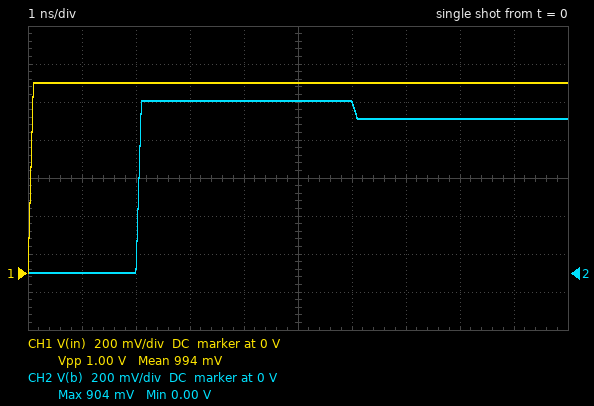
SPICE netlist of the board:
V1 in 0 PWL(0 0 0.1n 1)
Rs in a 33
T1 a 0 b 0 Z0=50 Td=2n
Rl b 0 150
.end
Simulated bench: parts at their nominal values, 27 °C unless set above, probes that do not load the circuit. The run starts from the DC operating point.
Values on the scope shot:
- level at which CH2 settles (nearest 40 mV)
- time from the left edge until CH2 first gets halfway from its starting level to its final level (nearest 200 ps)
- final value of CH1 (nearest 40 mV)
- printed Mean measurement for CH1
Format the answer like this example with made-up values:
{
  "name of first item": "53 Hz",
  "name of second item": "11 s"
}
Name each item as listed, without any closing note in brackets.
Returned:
{
  "level at which CH2 settles": "800 mV",
  "time from the left edge until CH2 first gets halfway from its starting level to its final level": "2.0 ns",
  "final value of CH1": "1.00 V",
  "printed Mean measurement for CH1": "994 mV"
}
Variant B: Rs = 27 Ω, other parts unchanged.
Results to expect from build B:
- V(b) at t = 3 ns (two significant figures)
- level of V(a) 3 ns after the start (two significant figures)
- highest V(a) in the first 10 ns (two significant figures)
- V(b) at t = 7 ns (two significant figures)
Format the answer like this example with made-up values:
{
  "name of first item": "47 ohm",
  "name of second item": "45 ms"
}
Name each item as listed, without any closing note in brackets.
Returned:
{
  "V(b) at t = 3 ns": "970 mV",
  "level of V(a) 3 ns after the start": "650 mV",
  "highest V(a) in the first 10 ns": "880 mV",
  "V(b) at t = 7 ns": "830 mV"
}
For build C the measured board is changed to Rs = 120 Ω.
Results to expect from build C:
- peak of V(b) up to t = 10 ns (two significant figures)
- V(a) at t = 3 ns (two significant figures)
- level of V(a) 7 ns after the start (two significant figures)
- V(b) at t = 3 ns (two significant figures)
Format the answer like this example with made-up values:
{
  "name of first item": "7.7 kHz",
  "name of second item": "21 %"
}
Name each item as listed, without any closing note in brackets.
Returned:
{
  "peak of V(b) up to t = 10 ns": "530 mV",
  "V(a) at t = 3 ns": "290 mV",
  "level of V(a) 7 ns after the start": "500 mV",
  "V(b) at t = 3 ns": "440 mV"
}
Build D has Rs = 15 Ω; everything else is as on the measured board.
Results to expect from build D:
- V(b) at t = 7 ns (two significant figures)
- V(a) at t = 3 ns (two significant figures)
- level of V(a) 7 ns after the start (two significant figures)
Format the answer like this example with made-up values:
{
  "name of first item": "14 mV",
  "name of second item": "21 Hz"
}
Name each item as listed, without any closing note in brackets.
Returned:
{
  "V(b) at t = 7 ns": "840 mV",
  "V(a) at t = 3 ns": "770 mV",
  "level of V(a) 7 ns after the start": "950 mV"
}
